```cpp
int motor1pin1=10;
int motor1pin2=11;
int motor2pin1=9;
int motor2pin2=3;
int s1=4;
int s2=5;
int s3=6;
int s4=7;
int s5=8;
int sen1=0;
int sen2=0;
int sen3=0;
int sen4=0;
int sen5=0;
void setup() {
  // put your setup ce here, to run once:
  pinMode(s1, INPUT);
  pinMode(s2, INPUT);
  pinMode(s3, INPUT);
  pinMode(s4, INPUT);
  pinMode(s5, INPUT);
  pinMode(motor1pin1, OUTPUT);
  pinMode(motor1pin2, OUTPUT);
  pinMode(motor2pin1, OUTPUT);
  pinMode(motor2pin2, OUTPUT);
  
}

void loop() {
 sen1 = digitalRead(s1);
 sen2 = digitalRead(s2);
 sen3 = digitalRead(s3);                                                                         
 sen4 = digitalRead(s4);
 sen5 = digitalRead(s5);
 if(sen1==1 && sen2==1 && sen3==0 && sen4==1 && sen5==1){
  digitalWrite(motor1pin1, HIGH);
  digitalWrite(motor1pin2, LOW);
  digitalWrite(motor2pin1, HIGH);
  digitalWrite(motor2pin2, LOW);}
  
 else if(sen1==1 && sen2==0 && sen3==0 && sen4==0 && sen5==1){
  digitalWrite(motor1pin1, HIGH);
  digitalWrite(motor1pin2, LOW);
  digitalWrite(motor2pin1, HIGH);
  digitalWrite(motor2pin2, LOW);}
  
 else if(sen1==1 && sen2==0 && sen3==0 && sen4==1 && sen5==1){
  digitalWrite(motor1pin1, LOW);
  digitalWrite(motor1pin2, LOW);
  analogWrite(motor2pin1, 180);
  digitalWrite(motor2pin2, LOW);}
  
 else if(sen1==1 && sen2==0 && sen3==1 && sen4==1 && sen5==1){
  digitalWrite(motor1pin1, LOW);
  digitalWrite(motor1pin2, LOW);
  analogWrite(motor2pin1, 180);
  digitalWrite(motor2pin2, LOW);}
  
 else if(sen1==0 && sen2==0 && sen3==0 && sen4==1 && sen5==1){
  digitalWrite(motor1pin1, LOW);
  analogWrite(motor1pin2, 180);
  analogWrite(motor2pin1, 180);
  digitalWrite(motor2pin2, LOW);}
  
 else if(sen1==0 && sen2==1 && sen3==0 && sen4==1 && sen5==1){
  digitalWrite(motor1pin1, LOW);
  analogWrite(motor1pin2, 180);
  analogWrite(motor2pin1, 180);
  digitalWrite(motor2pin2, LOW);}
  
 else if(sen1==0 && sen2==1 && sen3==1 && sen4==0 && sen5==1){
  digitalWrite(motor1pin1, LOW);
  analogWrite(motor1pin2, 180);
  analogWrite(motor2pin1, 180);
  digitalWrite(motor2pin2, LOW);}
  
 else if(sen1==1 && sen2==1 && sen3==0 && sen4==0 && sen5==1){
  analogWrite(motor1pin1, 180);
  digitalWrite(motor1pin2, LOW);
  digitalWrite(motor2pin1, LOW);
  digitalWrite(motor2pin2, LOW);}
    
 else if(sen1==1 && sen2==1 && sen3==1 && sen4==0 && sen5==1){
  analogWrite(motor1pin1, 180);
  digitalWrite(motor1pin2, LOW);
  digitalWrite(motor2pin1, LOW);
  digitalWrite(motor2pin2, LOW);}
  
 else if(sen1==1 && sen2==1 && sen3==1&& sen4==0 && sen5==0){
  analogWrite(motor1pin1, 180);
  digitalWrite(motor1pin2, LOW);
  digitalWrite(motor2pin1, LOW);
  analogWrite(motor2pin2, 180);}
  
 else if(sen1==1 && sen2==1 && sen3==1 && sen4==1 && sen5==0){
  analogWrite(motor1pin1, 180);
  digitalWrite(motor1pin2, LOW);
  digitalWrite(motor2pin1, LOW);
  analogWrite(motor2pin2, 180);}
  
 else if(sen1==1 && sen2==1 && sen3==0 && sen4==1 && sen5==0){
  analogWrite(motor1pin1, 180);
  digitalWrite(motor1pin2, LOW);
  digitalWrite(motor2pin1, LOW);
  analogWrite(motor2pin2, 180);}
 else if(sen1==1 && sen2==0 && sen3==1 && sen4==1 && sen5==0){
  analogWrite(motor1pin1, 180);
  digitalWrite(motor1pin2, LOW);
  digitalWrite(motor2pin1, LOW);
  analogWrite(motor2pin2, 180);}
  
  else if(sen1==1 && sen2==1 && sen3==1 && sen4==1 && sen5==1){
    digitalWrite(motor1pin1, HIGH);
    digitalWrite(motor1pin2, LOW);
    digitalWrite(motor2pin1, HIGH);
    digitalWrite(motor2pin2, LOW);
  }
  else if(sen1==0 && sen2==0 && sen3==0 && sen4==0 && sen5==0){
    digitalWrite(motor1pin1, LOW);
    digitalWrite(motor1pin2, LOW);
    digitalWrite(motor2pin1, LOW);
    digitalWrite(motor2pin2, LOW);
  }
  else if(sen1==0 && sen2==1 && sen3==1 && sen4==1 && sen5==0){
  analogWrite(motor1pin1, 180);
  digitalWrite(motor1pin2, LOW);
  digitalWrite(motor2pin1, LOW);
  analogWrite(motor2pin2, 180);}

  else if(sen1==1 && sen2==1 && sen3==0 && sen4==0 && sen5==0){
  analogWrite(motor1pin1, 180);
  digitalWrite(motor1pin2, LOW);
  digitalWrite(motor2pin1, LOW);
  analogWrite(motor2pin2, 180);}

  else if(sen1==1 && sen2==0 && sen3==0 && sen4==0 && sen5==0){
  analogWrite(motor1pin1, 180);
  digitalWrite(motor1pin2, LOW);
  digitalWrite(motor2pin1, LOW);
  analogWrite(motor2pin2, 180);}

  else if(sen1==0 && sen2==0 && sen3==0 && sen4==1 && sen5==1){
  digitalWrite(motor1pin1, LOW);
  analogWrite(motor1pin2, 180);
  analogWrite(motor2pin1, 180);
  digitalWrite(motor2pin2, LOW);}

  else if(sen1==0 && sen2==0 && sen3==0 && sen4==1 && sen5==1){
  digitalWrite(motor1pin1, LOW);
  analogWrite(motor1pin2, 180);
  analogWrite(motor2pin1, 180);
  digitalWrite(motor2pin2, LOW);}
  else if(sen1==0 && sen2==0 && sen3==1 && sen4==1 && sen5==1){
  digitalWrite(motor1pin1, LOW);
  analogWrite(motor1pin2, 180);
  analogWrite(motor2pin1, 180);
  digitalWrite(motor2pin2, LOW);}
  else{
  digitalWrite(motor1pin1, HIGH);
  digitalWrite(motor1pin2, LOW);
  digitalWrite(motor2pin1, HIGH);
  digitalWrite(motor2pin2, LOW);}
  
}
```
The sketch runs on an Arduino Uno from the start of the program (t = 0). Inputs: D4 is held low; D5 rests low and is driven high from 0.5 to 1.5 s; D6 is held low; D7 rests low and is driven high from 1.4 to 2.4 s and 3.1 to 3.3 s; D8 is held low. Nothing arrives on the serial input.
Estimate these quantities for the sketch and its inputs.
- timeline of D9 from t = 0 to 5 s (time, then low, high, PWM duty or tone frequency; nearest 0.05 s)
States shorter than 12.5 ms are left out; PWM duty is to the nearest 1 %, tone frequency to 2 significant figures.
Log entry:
0 s low; 0.5 s high; 2.4 s low; 3.1 s high; 3.3 s low
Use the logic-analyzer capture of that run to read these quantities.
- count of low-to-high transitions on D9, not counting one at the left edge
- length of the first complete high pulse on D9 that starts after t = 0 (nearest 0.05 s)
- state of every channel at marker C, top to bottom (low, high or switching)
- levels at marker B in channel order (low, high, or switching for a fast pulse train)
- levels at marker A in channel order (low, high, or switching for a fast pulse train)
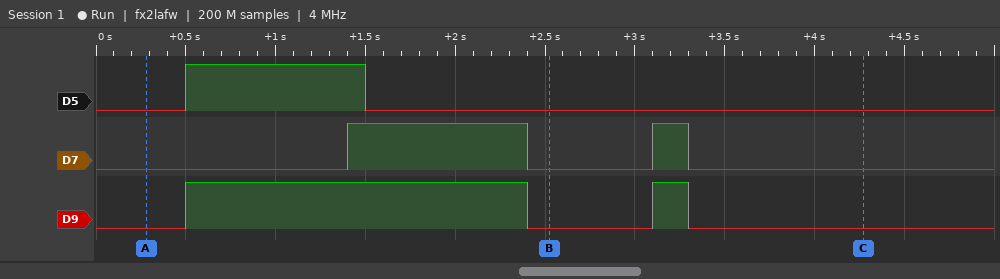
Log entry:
2
1.90 s
D5 low, D7 low, D9 low
D5 low, D7 low, D9 low
D5 low, D7 low, D9 low
